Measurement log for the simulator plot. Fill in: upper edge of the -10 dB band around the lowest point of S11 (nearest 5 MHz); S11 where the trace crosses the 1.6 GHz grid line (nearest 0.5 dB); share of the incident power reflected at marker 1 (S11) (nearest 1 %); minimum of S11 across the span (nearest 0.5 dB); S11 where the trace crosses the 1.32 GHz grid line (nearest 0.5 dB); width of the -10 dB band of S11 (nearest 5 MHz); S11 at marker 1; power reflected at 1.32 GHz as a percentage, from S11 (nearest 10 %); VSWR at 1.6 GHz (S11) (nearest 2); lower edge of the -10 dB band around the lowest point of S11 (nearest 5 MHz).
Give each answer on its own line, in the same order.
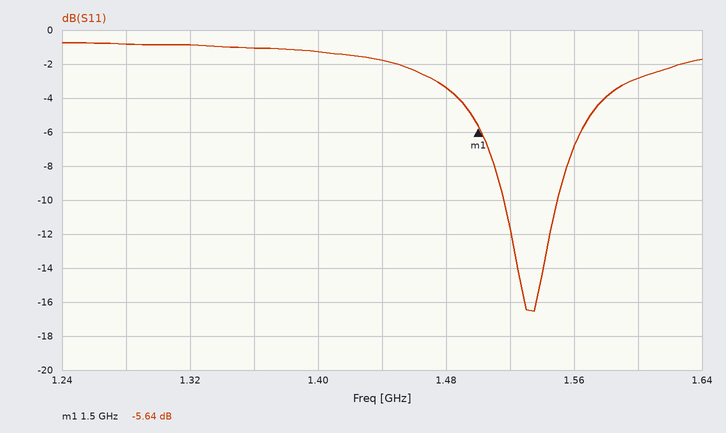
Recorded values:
1.550 GHz
-3.0 dB
27 %
-16.5 dB
-1.0 dB
35 MHz
-5.64 dB
80 %
6
1.515 GHz
